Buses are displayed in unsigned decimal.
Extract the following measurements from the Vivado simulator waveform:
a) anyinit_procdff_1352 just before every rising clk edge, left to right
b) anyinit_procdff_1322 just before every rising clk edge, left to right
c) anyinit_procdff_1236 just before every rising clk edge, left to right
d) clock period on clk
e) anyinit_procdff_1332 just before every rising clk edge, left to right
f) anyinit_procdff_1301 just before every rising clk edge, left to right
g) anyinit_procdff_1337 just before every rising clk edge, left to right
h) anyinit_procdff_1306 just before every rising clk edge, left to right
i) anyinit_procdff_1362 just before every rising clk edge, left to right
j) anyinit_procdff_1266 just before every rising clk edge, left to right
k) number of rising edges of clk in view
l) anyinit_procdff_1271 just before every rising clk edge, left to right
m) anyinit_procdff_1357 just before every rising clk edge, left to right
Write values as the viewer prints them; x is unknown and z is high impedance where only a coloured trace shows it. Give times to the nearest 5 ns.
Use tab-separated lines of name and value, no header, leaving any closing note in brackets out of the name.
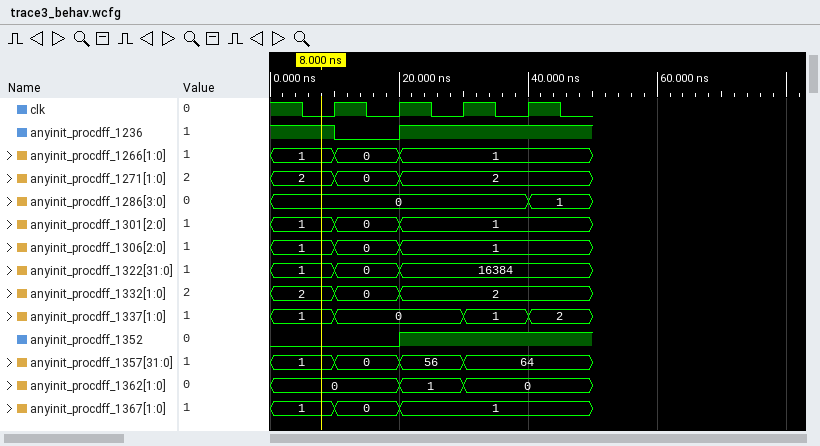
anyinit_procdff_1352 just before every rising clk edge, left to right	0 0 1 1
anyinit_procdff_1322 just before every rising clk edge, left to right	1, 0, 16384, 16384
anyinit_procdff_1236 just before every rising clk edge, left to right	1 0 1 1
clock period on clk	10 ns
anyinit_procdff_1332 just before every rising clk edge, left to right	2, 0, 2, 2
anyinit_procdff_1301 just before every rising clk edge, left to right	1, 0, 1, 1
anyinit_procdff_1337 just before every rising clk edge, left to right	1, 0, 0, 1
anyinit_procdff_1306 just before every rising clk edge, left to right	1, 0, 1, 1
anyinit_procdff_1362 just before every rising clk edge, left to right	0, 0, 1, 0
anyinit_procdff_1266 just before every rising clk edge, left to right	1, 0, 1, 1
number of rising edges of clk in view	4
anyinit_procdff_1271 just before every rising clk edge, left to right	2, 0, 2, 2
anyinit_procdff_1357 just before every rising clk edge, left to right	1, 0, 56, 64
